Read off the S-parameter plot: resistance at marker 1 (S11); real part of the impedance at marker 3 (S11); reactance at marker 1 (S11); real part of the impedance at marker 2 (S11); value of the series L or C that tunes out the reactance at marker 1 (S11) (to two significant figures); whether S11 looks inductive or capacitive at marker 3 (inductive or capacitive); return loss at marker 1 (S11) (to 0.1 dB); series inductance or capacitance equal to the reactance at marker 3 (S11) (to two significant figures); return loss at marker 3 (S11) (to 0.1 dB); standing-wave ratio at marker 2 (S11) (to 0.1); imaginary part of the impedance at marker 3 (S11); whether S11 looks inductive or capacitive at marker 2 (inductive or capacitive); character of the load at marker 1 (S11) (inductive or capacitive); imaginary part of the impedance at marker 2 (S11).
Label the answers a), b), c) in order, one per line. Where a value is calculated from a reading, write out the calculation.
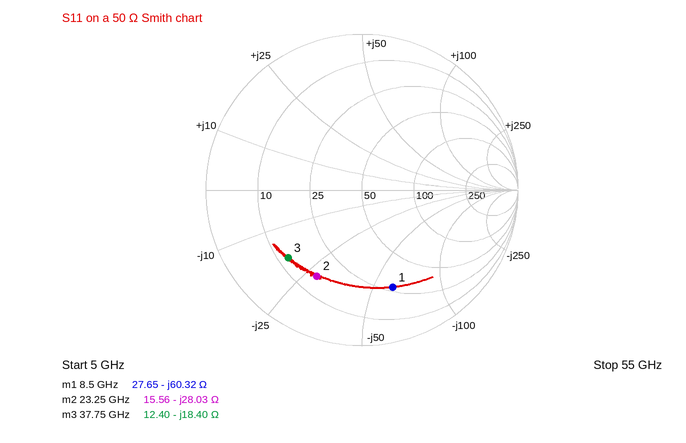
a) 27.65 Ω
b) 12.40 Ω
c) -60.32 Ω
d) 15.56 Ω
e) L = 60.32 Ω/(2π × 8.5 GHz) ≈ 1.1 nH
f) capacitive
g) 3.7 dB
h) C = 1/(2π × 37.75 GHz × 18.4 Ω) ≈ 229 fF, so 230 fF to two significant figures
i) 3.8 dB
j) 4.3
k) -18.40 Ω
l) capacitive
m) capacitive
n) -28.03 Ω
